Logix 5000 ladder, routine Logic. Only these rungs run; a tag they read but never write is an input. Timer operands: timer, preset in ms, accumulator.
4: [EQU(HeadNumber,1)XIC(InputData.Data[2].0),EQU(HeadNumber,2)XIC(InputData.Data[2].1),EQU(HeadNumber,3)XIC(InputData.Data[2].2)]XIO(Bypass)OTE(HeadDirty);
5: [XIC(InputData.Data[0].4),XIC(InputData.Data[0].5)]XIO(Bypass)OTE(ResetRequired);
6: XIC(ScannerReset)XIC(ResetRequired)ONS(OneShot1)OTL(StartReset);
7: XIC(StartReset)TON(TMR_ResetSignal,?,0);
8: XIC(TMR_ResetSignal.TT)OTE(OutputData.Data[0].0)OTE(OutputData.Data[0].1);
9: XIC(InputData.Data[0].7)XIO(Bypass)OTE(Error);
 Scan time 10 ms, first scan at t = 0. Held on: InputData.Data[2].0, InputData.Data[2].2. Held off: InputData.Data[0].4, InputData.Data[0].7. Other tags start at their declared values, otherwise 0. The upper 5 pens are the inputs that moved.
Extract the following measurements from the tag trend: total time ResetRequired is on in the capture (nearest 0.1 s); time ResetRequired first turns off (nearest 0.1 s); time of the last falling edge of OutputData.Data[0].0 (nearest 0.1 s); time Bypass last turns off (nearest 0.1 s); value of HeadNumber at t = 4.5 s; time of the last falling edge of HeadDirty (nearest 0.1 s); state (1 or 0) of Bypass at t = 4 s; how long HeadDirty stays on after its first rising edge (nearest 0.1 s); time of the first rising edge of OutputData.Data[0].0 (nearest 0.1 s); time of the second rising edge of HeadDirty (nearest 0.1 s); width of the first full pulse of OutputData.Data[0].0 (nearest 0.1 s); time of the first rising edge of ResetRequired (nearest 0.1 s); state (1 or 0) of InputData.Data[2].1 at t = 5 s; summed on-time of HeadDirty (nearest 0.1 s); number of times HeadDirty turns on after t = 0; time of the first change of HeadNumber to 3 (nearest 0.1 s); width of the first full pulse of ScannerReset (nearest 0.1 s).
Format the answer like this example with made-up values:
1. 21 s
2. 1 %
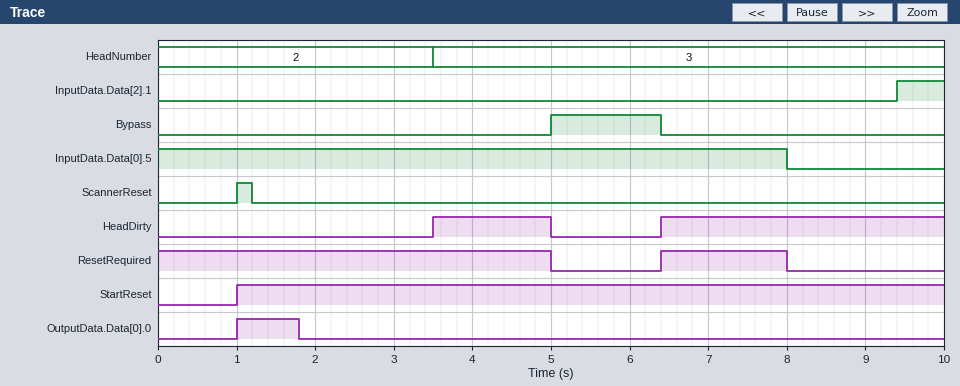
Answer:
1. 6.6 s
2. 5.0 s
3. 1.8 s
4. 6.4 s
5. 3
6. 5.0 s
7. 0
8. 1.5 s
9. 1.0 s
10. 6.4 s
11. 0.8 s
12. 6.4 s
13. 0
14. 5.1 s
15. 2
16. 3.5 s
17. 0.2 s
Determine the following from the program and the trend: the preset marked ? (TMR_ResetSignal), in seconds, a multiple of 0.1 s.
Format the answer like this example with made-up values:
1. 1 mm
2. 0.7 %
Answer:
1. 0.8 s
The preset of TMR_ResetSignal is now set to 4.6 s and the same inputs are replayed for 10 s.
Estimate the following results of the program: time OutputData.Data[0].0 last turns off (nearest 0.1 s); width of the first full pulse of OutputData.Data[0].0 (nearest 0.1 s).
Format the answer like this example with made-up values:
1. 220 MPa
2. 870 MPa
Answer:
1. 5.6 s
2. 4.6 s
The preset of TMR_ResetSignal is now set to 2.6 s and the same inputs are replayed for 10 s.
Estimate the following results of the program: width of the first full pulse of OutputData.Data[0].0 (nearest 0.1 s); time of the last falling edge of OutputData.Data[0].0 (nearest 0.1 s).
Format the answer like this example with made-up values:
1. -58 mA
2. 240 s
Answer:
1. 2.6 s
2. 3.6 s
